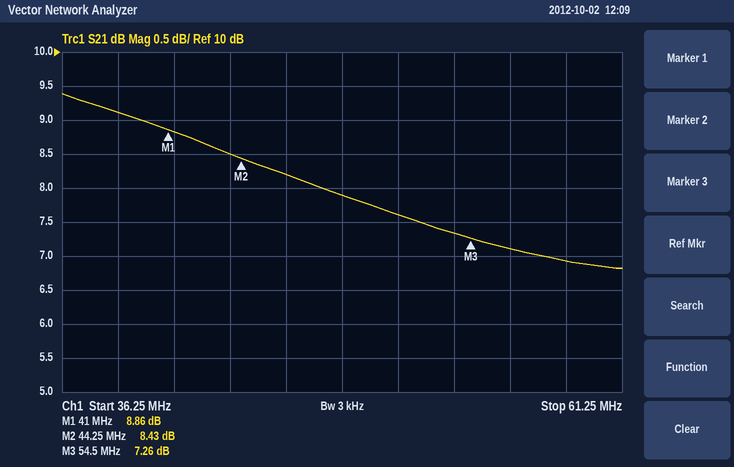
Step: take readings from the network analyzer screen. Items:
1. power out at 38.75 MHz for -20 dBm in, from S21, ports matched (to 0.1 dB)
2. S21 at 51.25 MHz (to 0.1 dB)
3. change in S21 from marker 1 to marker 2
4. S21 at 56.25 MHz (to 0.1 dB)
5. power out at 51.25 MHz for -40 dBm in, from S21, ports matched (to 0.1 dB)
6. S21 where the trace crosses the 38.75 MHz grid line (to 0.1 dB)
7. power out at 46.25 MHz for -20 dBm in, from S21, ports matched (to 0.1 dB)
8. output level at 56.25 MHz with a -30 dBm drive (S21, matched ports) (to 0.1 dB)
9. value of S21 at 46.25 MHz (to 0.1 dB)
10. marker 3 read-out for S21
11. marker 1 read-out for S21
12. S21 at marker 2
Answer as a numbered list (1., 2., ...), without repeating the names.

1. -10.9 dBm
2. 7.6 dB
3. -0.43 dB
4. 7.1 dB
5. -32.4 dBm
6. 9.1 dB
7. -11.8 dBm
8. -22.9 dBm
9. 8.2 dB
10. 7.26 dB
11. 8.86 dB
12. 8.43 dB
